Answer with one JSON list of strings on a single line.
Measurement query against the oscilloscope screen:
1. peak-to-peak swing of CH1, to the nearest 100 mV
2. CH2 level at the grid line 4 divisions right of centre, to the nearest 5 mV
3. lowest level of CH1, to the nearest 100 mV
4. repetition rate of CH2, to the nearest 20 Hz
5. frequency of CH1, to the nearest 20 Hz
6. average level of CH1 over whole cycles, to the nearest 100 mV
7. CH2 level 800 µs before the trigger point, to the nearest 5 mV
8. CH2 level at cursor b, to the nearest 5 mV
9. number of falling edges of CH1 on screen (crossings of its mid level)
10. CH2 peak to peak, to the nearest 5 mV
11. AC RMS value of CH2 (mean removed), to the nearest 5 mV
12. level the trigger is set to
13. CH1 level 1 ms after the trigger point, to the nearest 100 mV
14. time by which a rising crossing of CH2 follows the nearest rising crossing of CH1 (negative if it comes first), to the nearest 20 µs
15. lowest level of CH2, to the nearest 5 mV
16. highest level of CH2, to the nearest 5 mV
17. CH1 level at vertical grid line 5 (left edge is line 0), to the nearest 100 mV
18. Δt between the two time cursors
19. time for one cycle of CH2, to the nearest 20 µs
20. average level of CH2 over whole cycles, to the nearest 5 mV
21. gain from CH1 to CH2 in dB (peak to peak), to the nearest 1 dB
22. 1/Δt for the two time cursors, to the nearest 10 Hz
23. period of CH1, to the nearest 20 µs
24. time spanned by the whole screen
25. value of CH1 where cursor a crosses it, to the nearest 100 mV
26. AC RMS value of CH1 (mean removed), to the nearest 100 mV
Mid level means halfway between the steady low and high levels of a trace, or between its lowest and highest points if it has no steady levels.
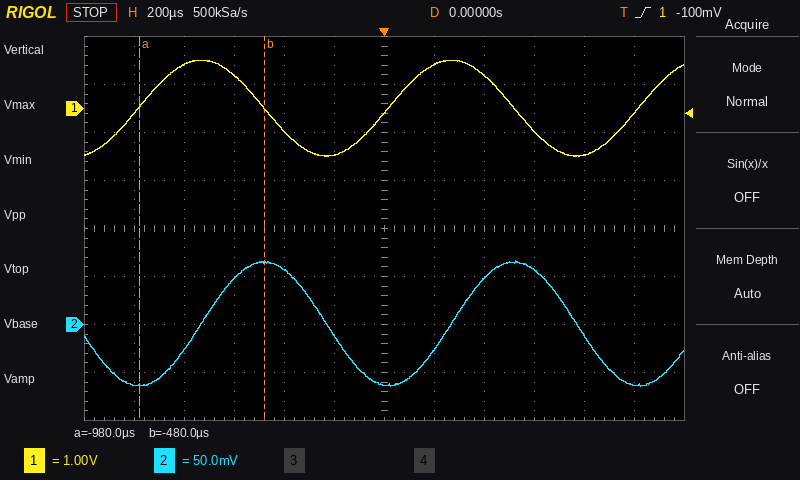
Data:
["2.0 V", "-10 mV", "-1.0 V", "1.00 kHz", "1.00 kHz", "0.0 V", "-25 mV", "65 mV", "2", "130 mV", "45 mV", "-100 mV", "-100 mV", "+260 µs", "-65 mV", "65 mV", "-1.0 V", "500 µs", "1.00 ms", "0 mV", "-24 dB", "2.00 kHz", "1.00 ms", "2.4 ms", "0.0 V", "700 mV"]
